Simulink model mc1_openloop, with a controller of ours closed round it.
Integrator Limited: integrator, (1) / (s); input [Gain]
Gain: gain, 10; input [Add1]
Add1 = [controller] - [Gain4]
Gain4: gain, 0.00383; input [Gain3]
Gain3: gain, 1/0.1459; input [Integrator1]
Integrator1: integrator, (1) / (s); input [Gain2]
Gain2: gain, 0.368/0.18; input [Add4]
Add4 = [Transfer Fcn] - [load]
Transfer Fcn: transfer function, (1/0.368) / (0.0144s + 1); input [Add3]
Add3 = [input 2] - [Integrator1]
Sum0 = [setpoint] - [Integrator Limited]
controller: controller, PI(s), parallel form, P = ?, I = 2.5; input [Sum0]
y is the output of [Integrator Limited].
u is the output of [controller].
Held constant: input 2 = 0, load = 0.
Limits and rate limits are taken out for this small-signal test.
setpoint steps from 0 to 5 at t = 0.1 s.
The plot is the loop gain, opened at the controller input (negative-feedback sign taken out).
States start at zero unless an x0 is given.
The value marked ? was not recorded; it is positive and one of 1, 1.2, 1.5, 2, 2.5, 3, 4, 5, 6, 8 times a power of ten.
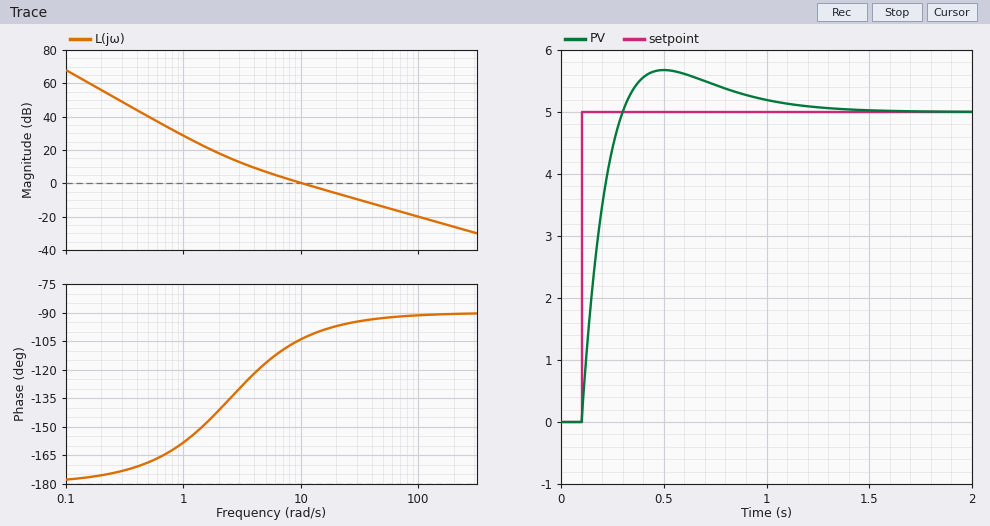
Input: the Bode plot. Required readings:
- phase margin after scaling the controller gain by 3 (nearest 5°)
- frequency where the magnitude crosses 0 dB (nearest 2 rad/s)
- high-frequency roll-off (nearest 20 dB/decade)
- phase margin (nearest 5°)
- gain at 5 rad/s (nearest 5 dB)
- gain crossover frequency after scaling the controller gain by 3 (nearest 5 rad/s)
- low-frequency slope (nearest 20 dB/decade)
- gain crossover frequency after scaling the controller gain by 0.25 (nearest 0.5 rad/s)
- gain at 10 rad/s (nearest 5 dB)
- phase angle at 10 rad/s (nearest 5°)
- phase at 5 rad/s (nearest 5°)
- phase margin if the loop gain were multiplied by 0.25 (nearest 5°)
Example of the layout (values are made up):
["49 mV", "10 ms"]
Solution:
["85°", "10 rad/s", "-20 dB/decade", "75°", "5 dB", "30 rad/s", "-40 dB/decade", "3.0 rad/s", "0 dB", "-105°", "-115°", "50°"]
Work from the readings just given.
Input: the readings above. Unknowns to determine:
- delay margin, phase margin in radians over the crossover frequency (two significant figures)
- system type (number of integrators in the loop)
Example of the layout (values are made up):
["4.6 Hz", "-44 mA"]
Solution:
["0.13 s", "2"]
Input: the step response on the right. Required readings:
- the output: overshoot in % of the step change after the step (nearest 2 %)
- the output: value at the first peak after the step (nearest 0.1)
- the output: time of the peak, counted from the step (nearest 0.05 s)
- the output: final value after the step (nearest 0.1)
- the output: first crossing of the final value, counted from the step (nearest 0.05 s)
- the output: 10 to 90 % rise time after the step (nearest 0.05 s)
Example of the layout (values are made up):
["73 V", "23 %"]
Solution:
["14 %", "5.7", "0.40 s", "5.0", "0.20 s", "0.15 s"]
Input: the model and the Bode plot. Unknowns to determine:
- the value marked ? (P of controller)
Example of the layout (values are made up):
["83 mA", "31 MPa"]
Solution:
["1"]
